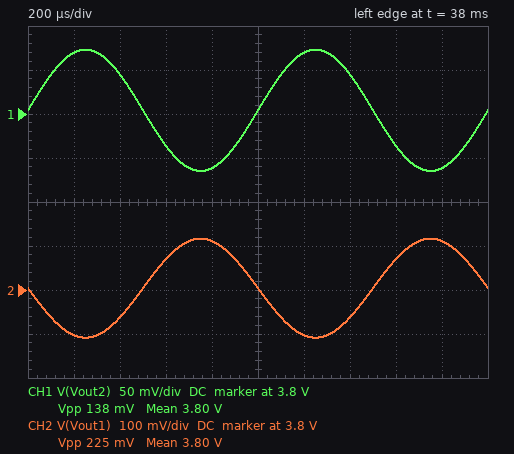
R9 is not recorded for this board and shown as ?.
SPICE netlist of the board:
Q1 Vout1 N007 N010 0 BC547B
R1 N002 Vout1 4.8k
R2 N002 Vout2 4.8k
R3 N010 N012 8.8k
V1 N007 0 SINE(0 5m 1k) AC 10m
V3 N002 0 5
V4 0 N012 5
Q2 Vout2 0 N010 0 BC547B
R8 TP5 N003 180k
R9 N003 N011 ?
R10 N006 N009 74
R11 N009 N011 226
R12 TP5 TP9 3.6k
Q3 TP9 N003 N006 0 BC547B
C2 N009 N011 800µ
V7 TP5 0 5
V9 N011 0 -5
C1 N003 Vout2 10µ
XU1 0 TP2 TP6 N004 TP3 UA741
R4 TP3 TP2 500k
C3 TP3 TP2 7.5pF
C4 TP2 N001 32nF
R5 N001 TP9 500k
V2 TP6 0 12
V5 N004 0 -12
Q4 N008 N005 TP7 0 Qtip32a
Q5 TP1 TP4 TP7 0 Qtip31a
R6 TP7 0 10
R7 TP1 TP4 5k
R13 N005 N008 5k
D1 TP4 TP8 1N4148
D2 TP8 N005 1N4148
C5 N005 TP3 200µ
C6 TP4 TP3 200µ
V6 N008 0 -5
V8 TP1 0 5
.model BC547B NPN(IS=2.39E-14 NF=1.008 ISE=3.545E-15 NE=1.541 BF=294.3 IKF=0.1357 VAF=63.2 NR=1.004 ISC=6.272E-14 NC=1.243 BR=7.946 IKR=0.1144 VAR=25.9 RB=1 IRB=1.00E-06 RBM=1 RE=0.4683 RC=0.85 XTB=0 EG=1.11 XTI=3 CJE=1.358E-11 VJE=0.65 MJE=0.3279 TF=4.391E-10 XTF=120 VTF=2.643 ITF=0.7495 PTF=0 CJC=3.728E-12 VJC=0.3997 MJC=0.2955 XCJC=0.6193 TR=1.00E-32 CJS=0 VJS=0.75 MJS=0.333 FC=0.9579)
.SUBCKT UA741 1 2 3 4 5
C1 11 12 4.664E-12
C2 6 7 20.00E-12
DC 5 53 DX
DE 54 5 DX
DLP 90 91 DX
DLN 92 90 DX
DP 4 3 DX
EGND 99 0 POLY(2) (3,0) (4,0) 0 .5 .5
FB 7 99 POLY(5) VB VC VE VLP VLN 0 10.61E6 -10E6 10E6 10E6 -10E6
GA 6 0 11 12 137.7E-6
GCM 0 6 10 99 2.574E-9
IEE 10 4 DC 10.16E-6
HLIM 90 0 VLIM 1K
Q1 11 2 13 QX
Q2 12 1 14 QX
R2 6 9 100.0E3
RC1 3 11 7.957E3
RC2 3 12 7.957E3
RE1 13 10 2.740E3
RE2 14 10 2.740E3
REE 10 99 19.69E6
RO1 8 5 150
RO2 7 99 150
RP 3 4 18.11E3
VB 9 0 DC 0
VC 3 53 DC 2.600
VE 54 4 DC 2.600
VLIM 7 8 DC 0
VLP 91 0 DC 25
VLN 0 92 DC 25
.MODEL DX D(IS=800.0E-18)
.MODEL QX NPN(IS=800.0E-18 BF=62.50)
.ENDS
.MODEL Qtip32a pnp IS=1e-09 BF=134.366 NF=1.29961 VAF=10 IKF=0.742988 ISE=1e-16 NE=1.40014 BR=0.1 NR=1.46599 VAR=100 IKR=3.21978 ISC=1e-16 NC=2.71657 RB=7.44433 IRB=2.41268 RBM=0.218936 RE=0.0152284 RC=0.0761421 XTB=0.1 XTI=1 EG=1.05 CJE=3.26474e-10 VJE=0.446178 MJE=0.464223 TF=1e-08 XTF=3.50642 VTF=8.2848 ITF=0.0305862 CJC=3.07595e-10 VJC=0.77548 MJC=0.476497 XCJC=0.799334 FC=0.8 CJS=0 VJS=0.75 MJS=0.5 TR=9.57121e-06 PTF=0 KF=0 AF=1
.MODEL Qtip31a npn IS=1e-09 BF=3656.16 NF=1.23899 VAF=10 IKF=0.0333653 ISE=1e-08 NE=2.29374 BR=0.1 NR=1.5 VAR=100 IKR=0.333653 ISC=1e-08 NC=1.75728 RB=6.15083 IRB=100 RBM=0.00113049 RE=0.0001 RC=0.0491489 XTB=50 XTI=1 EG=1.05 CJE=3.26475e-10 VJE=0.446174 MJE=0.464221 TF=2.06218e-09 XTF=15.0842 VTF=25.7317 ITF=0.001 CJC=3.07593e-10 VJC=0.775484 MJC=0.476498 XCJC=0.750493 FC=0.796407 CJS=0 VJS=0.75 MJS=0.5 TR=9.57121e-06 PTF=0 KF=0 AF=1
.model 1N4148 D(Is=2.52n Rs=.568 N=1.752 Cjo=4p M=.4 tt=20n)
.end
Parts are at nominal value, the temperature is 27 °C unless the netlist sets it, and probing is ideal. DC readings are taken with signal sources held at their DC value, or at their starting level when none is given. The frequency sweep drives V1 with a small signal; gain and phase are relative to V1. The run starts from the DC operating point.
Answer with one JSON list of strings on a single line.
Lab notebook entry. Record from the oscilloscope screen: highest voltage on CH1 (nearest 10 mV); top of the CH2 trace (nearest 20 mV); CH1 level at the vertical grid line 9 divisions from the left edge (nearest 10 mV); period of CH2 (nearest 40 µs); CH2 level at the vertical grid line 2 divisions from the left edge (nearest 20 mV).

["3.87 V", "3.92 V", "3.74 V", "1.00 ms", "3.74 V"]
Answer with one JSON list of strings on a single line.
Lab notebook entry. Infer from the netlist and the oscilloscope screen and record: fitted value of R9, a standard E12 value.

["8.2 kΩ"]
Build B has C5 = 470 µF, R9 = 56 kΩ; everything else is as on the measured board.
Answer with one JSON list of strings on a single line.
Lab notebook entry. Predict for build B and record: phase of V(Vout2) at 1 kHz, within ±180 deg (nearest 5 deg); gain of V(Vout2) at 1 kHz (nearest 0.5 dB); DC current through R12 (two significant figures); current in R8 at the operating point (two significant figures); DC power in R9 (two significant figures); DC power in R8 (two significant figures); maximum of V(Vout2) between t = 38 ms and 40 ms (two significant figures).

["-5 deg", "-1.5 dB", "2.5 mA", "48 µA", "37 µW", "410 µW", "3.8 V"]
